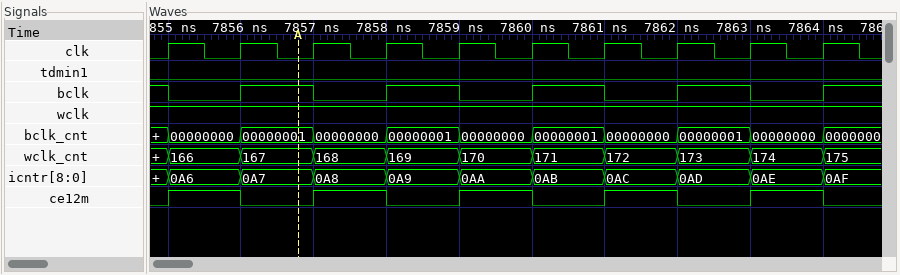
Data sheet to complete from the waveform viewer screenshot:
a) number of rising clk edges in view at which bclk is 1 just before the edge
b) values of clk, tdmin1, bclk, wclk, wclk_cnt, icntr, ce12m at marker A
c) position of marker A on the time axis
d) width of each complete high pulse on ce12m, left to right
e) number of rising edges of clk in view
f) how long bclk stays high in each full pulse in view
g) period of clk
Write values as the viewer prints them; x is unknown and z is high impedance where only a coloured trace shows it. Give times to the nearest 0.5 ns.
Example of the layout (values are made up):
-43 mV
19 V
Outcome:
5
clk=0, tdmin1=0, bclk=1, wclk=1, wclk_cnt=167, icntr=0A7, ce12m=0
7857 ns
1 ns, 1 ns, 1 ns, 1 ns, 1 ns
10
1 ns, 1 ns, 1 ns, 1 ns
1 ns
